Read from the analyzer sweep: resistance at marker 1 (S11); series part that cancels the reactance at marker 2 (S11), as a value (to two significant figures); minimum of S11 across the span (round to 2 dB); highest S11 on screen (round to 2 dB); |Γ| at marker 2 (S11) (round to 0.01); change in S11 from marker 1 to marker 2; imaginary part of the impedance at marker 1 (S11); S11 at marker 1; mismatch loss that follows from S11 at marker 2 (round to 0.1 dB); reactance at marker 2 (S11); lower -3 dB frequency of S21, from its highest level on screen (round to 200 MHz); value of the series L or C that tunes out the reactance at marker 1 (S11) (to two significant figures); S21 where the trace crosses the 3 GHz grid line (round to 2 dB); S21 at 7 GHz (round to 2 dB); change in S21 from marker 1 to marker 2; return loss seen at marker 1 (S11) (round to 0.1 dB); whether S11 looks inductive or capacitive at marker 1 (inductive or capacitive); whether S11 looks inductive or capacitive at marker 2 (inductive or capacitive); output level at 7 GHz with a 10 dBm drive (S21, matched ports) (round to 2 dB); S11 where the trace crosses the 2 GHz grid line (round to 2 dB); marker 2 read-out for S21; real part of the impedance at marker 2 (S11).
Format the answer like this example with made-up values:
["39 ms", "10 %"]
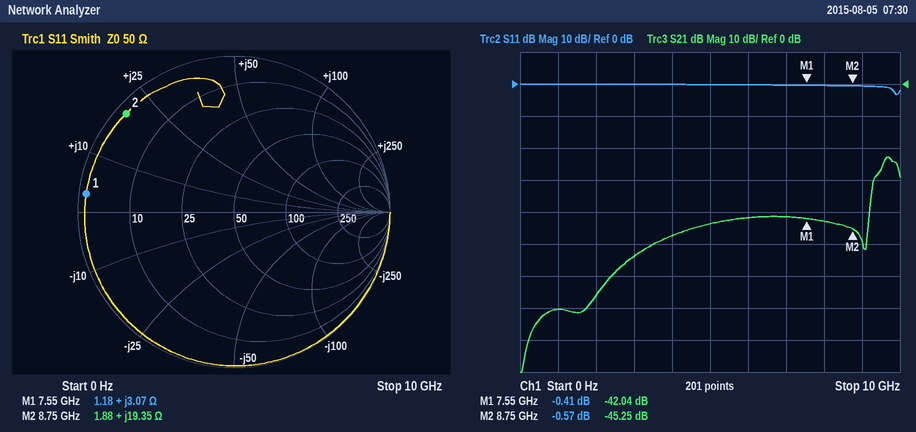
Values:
["1.18 Ω", "940 fF", "-4 dB", "0 dB", "0.94", "-0.16 dB", "+3.07 Ω", "-0.41 dB", "9.1 dB", "+19.35 Ω", "9.6 GHz", "6.9 pF", "-54 dB", "-42 dB", "-3.21 dB", "0.4 dB", "inductive", "inductive", "-32 dBm", "0 dB", "-45.25 dB", "1.88 Ω"]
